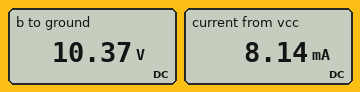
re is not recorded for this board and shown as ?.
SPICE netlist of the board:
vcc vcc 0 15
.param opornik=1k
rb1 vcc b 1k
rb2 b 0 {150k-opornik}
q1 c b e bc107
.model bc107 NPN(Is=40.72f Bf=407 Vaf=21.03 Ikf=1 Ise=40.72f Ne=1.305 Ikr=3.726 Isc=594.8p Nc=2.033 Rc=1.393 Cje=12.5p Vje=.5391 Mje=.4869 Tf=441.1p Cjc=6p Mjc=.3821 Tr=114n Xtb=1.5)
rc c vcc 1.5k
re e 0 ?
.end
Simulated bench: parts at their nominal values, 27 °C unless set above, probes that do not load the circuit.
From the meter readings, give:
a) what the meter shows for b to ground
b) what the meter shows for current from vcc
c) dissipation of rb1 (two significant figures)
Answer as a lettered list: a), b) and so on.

a) 10.37 V
b) 8.14 mA
c) 21 mW
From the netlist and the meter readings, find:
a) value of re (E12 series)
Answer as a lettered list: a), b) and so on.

a) 1.2 kΩ
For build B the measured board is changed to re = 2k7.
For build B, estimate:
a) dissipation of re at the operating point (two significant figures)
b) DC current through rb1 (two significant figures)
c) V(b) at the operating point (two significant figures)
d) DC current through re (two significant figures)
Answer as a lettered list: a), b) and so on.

a) 52 mW
b) 2.4 mA
c) 13 V
d) 4.4 mA
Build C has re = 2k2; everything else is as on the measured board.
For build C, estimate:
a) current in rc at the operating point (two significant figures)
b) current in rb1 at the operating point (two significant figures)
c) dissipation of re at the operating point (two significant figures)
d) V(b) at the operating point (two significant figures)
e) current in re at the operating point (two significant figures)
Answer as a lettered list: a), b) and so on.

a) 2.4 mA
b) 2.9 mA
c) 59 mW
d) 12 V
e) 5.2 mA
